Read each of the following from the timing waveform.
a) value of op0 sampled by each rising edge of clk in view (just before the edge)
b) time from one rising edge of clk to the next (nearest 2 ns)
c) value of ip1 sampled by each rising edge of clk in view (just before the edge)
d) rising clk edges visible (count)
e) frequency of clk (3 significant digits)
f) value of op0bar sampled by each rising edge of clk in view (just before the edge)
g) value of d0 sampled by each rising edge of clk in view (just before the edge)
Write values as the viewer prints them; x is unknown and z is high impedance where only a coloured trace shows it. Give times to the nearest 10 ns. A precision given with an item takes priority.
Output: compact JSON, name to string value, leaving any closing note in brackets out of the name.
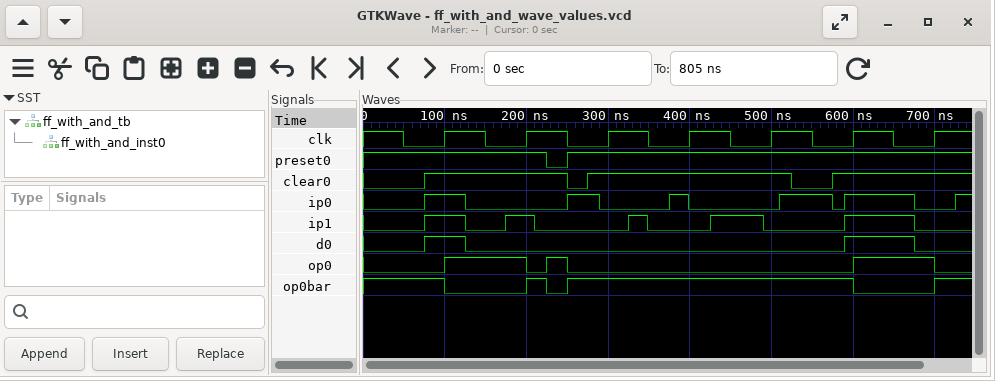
{"value of op0 sampled by each rising edge of clk in view": "0 1 0 0 0 0 1", "time from one rising edge of clk to the next": "100 ns", "value of ip1 sampled by each rising edge of clk in view": "1 1 0 0 0 1 0", "rising clk edges visible": "7", "frequency of clk": "10.0 MHz", "value of op0bar sampled by each rising edge of clk in view": "1 0 1 1 1 1 0", "value of d0 sampled by each rising edge of clk in view": "1 0 0 0 0 1 0"}
